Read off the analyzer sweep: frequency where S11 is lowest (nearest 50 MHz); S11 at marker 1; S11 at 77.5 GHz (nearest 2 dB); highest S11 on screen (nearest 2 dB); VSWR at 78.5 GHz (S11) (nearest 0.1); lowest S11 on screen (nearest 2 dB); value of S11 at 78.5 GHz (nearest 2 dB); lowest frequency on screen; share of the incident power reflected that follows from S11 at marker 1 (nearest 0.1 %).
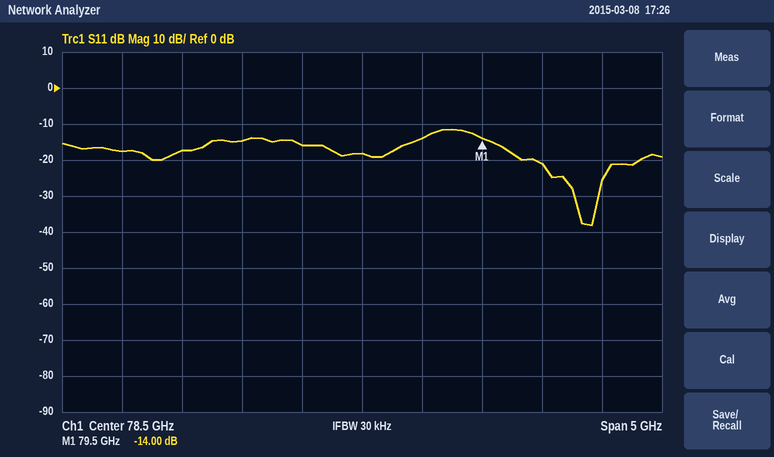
80.40 GHz
-14.00 dB
-14 dB
-12 dB
1.3
-38 dB
-18 dB
76 GHz
4.0 %
